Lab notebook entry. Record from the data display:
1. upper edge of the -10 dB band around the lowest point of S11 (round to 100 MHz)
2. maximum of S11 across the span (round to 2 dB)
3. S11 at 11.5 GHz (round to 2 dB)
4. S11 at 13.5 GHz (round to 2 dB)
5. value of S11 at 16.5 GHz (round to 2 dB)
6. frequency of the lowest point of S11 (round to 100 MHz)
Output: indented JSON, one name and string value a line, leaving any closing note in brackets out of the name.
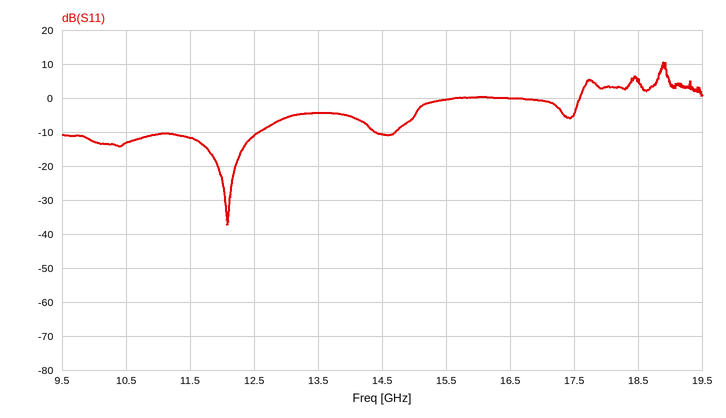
{
  "upper edge of the -10 dB band around the lowest point of S11": "12.6 GHz",
  "maximum of S11 across the span": "10 dB",
  "S11 at 11.5 GHz": "-12 dB",
  "S11 at 13.5 GHz": "-4 dB",
  "value of S11 at 16.5 GHz": "0 dB",
  "frequency of the lowest point of S11": "12.1 GHz"
}
